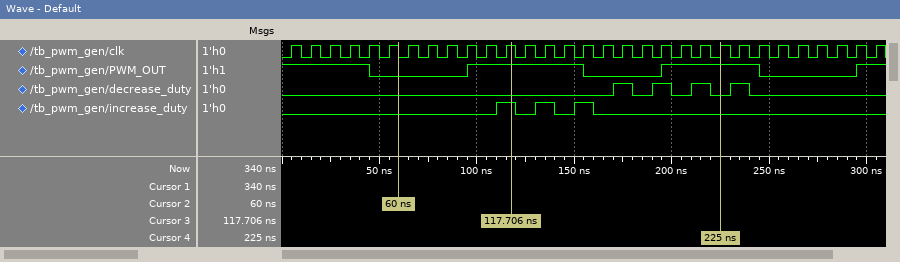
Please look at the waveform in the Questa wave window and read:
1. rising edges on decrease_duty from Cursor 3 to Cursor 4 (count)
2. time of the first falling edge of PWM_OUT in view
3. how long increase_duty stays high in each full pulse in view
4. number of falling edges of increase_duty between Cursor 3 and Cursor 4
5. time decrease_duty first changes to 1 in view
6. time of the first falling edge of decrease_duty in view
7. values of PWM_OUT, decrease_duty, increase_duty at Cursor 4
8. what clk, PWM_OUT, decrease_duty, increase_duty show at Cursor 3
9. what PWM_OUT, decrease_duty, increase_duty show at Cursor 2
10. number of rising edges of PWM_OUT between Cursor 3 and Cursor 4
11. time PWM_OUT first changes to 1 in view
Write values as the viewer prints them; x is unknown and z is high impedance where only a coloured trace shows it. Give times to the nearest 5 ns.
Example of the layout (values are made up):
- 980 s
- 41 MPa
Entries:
- 3
- 45 ns
- 10 ns, 10 ns, 10 ns
- 3
- 170 ns
- 180 ns
- PWM_OUT=1, decrease_duty=0, increase_duty=0
- clk=1, PWM_OUT=1, decrease_duty=0, increase_duty=1
- PWM_OUT=0, decrease_duty=0, increase_duty=0
- 1
- 95 ns
